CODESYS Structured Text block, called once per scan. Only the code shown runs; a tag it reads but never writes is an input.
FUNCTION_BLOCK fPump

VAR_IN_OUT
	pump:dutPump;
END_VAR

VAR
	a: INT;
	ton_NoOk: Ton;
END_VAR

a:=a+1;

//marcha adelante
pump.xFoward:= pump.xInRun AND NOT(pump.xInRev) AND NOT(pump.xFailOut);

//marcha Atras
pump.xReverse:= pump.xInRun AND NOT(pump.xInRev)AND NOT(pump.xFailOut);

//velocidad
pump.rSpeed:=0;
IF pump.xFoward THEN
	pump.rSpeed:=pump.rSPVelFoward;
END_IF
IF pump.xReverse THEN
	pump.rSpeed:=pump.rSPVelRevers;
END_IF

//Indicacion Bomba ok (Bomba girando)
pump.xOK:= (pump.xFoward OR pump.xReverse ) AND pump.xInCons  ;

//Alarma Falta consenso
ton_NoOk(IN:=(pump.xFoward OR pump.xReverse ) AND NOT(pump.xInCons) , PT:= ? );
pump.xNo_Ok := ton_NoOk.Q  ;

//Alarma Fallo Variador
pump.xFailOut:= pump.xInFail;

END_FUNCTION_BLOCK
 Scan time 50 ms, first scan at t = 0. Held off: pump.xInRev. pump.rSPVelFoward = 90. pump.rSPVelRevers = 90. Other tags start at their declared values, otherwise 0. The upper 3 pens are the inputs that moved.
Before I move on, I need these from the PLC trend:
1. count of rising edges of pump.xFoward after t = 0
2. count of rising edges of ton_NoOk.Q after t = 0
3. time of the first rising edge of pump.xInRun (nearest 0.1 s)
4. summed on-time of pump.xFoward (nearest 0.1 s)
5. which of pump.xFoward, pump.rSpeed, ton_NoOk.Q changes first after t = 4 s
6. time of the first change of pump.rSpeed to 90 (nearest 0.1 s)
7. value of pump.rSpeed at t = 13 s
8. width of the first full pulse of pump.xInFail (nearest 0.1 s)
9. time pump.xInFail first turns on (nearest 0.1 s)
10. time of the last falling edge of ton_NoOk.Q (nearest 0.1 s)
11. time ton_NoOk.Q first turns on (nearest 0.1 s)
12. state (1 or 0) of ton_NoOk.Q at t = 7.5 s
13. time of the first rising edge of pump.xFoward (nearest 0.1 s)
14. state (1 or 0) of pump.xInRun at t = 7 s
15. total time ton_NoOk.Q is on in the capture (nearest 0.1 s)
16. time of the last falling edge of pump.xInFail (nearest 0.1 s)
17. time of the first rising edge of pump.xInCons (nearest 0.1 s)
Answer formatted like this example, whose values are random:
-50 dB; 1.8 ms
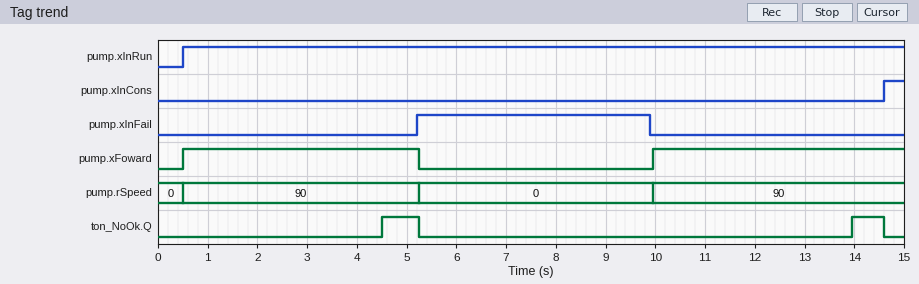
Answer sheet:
2; 2; 0.5 s; 9.8 s; ton_NoOk.Q; 0.5 s; 90; 4.7 s; 5.2 s; 14.6 s; 4.5 s; 0; 0.5 s; 1; 1.4 s; 9.9 s; 14.6 s
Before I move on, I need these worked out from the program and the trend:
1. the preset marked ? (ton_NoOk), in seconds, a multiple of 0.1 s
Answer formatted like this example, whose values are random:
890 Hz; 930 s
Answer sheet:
4.0 s
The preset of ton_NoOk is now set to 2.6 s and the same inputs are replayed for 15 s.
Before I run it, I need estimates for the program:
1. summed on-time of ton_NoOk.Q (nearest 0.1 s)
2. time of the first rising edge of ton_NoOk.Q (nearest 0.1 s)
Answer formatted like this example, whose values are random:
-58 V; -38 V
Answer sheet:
4.2 s; 3.1 s
